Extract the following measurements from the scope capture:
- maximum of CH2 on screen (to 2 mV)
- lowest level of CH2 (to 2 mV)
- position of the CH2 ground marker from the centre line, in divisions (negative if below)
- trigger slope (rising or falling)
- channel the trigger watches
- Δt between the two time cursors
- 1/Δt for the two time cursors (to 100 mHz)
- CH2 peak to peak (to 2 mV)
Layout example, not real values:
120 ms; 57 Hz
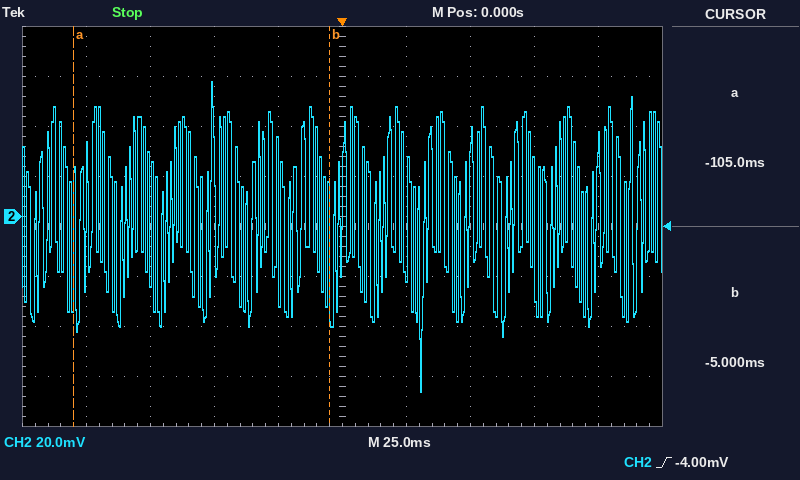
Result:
54 mV; -70 mV; +0.2 div; rising; CH2; 100.0 ms; 10.0 Hz; 124 mV
